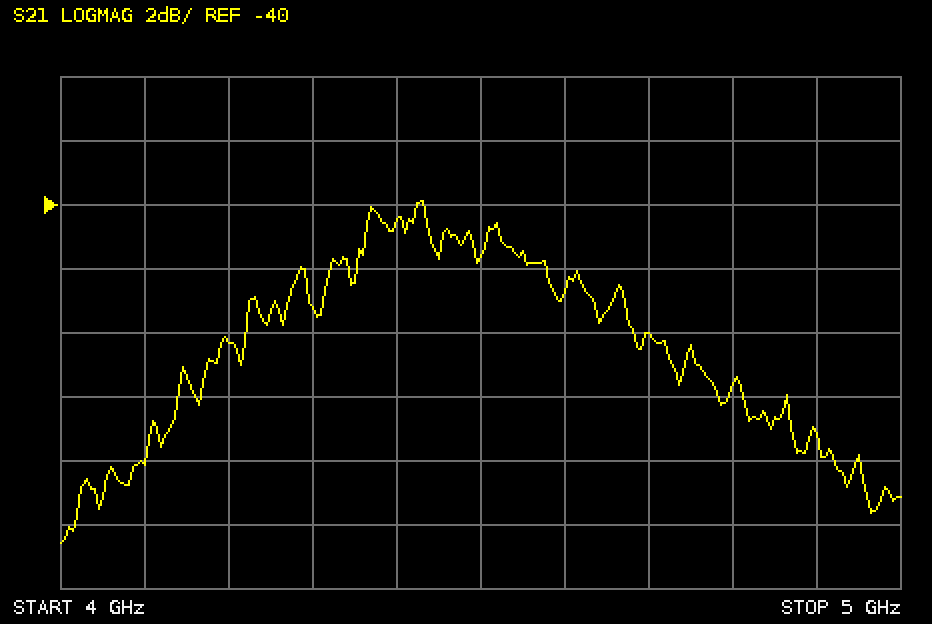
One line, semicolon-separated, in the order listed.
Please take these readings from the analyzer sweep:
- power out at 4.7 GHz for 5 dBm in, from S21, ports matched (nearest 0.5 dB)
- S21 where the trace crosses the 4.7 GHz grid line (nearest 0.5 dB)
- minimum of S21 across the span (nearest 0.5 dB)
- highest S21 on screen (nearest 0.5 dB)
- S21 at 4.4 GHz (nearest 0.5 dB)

-39.0 dBm; -44.0 dB; -50.5 dB; -40.0 dB; -40.5 dB
